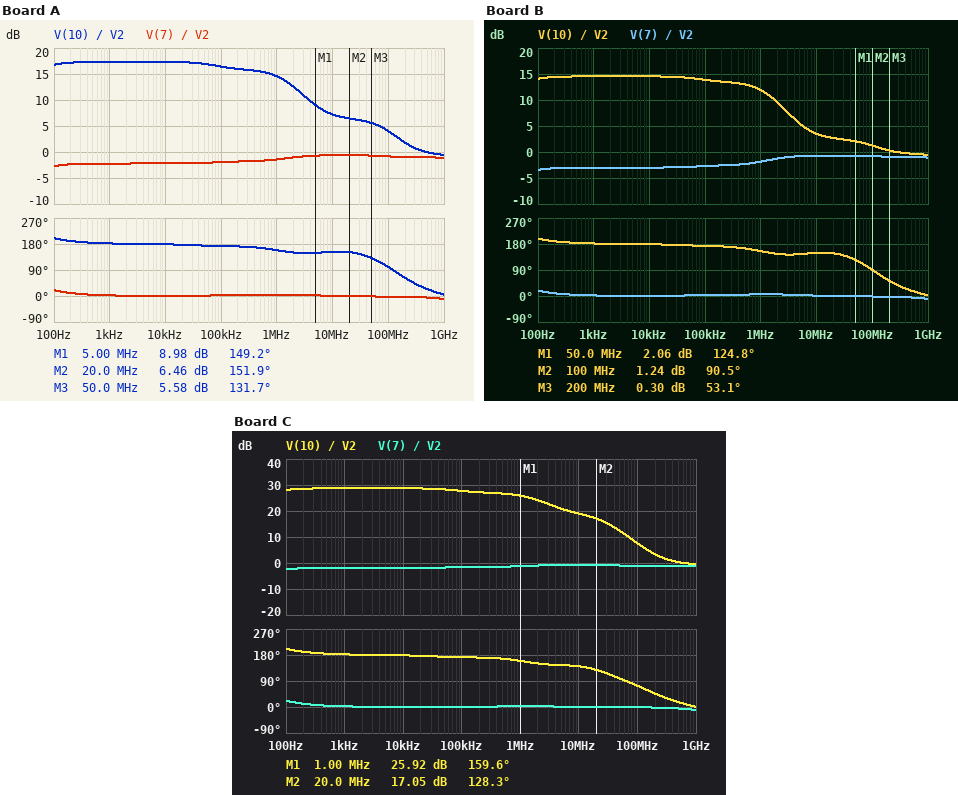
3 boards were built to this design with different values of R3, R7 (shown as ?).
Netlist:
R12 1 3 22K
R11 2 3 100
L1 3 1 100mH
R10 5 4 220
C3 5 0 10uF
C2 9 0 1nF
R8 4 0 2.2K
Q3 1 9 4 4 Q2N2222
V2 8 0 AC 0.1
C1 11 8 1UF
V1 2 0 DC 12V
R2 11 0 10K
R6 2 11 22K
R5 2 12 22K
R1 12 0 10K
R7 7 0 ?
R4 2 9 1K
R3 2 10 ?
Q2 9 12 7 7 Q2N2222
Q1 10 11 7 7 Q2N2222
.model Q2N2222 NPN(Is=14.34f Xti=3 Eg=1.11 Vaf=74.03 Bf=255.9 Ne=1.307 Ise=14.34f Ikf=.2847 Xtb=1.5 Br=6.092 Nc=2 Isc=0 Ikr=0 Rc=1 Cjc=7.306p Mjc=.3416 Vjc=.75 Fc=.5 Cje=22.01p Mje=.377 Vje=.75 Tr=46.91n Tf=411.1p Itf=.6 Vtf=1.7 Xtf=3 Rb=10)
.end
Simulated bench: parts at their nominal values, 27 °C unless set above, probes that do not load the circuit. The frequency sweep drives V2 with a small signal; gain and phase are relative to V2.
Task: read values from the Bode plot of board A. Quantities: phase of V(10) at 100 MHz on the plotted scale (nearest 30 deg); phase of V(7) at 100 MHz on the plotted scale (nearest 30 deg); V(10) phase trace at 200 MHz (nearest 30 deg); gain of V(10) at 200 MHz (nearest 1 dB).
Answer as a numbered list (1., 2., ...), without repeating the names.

1. 90 deg
2. 0 deg
3. 60 deg
4. 2 dB
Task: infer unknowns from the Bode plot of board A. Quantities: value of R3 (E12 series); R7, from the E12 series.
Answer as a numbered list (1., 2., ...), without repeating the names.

1. 470 Ω
2. 820 Ω
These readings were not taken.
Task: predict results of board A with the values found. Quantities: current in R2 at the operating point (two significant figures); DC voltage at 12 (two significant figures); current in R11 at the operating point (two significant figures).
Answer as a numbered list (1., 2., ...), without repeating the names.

1. 370 µA
2. 3.7 V
3. 4.3 mA
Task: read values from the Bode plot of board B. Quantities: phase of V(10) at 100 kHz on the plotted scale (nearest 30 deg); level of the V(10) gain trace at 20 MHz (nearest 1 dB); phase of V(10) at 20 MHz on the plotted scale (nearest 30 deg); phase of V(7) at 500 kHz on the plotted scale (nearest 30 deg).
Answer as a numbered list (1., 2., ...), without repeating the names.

1. 180 deg
2. 3 dB
3. 150 deg
4. 0 deg
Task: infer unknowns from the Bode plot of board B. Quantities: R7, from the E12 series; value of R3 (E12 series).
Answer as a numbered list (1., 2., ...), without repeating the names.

1. 1.5 kΩ
2. 470 Ω
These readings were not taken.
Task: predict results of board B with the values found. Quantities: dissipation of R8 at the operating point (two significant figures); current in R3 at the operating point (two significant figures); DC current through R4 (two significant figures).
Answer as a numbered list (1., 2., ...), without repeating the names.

1. 48 mW
2. 1.0 mA
3. 1.0 mA
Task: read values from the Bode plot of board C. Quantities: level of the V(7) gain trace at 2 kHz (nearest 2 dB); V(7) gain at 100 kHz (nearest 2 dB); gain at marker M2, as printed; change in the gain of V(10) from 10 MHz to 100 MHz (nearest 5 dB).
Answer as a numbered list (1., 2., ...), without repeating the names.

1. -2 dB
2. -2 dB
3. 17.05 dB
4. -10 dB
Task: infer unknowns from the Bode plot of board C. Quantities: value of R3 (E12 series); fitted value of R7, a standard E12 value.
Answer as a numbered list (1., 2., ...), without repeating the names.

1. 1.5 kΩ
2. 560 Ω
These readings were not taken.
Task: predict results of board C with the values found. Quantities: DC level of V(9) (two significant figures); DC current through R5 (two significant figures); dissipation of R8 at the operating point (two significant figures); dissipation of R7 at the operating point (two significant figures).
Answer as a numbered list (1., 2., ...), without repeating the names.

1. 9.3 V
2. 380 µA
3. 34 mW
4. 16 mW
